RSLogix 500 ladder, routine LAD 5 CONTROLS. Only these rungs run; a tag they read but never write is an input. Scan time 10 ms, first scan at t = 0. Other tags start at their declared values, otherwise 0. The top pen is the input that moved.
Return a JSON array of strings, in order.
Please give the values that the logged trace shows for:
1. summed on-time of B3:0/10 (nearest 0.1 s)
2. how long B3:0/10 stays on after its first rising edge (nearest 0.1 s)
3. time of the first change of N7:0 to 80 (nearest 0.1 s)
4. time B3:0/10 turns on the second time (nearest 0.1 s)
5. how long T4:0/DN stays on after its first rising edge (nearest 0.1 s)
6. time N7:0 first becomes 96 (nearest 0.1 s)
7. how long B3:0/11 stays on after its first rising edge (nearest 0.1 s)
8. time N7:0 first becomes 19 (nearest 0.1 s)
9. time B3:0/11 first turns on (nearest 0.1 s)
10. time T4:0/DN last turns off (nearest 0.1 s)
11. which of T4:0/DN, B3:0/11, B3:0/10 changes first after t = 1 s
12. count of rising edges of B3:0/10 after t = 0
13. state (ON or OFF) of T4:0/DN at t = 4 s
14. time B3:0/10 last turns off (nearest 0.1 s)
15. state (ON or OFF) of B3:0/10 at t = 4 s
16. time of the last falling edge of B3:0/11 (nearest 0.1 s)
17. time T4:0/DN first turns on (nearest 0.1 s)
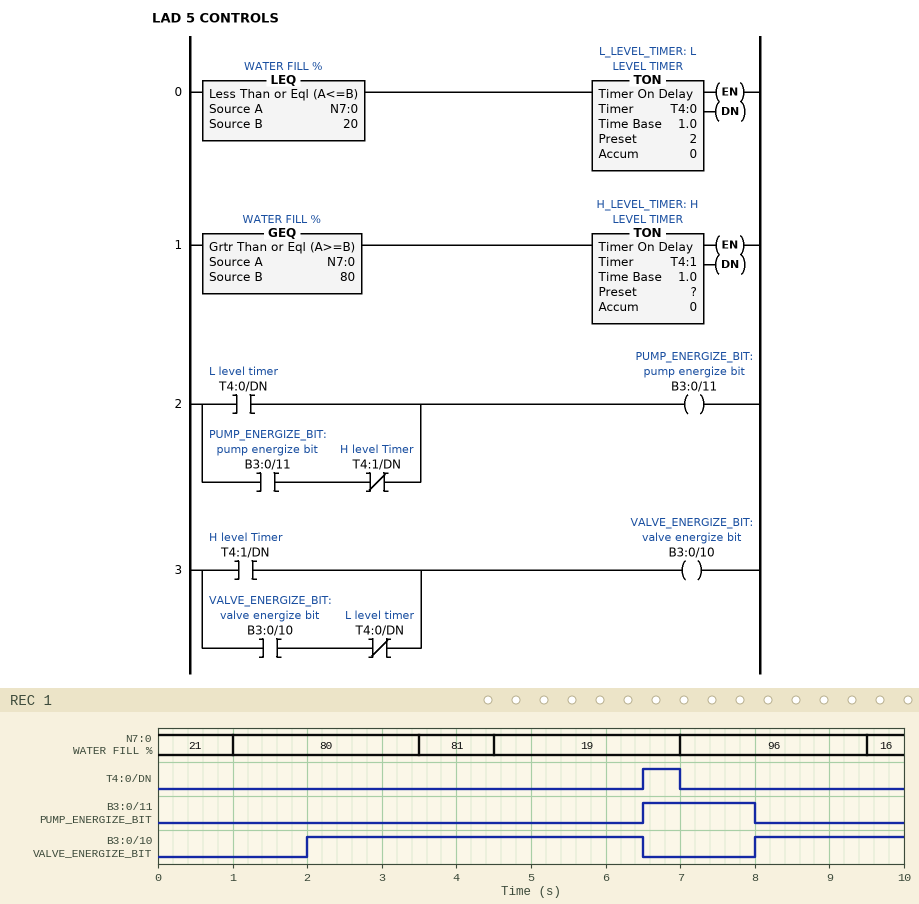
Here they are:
["6.5 s", "4.5 s", "1.0 s", "8.0 s", "0.5 s", "7.0 s", "1.5 s", "4.5 s", "6.5 s", "7.0 s", "B3:0/10", "2", "OFF", "6.5 s", "ON", "8.0 s", "6.5 s"]
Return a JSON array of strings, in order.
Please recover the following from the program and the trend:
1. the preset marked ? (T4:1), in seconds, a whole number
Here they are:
["1 s"]
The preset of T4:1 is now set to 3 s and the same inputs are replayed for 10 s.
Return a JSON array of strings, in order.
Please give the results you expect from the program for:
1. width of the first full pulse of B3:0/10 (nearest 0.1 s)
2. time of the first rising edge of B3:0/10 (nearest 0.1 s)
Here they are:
["2.5 s", "4.0 s"]
